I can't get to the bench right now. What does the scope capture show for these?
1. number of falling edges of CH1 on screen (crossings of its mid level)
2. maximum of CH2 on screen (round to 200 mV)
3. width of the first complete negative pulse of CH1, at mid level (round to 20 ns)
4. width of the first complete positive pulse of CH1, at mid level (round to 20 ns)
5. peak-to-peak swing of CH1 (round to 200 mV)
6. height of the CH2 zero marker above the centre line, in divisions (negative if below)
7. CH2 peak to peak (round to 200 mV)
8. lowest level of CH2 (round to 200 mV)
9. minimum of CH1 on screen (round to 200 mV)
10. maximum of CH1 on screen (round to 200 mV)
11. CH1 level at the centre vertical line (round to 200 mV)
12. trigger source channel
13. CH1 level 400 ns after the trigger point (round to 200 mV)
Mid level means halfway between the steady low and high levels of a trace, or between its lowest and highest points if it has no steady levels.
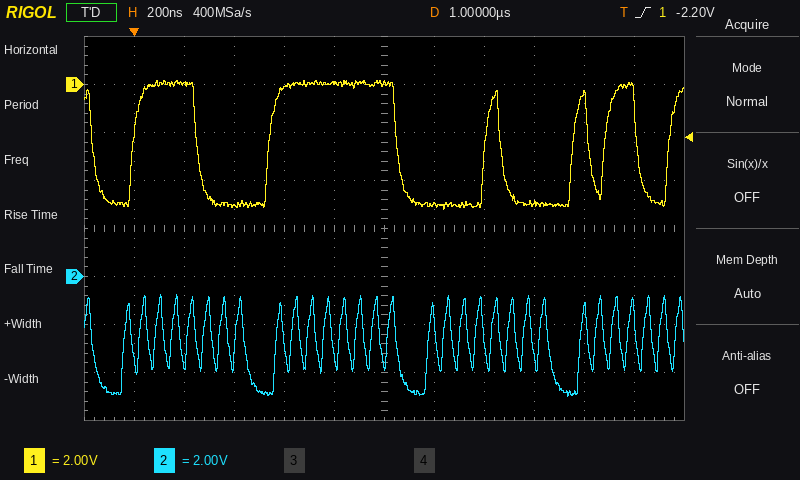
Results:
6
-800 mV
160 ns
260 ns
5.4 V
-1.0 div
4.2 V
-5.0 V
-5.2 V
200 mV
0.0 V
CH1
-5.0 V
